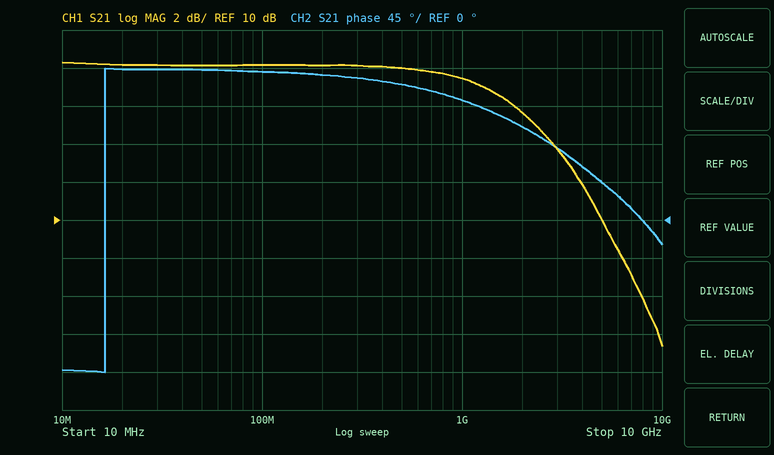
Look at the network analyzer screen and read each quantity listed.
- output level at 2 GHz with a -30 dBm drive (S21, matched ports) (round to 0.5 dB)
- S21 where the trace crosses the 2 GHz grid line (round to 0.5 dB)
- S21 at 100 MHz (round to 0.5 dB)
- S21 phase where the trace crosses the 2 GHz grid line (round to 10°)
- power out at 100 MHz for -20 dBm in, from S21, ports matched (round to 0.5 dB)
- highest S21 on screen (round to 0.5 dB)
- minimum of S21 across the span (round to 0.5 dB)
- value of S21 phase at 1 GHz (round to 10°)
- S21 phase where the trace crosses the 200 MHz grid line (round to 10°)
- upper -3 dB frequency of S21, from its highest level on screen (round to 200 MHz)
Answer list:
-14.5 dBm
15.5 dB
18.0 dB
110°
-2.0 dBm
18.5 dB
3.5 dB
140°
170°
2.2 GHz
